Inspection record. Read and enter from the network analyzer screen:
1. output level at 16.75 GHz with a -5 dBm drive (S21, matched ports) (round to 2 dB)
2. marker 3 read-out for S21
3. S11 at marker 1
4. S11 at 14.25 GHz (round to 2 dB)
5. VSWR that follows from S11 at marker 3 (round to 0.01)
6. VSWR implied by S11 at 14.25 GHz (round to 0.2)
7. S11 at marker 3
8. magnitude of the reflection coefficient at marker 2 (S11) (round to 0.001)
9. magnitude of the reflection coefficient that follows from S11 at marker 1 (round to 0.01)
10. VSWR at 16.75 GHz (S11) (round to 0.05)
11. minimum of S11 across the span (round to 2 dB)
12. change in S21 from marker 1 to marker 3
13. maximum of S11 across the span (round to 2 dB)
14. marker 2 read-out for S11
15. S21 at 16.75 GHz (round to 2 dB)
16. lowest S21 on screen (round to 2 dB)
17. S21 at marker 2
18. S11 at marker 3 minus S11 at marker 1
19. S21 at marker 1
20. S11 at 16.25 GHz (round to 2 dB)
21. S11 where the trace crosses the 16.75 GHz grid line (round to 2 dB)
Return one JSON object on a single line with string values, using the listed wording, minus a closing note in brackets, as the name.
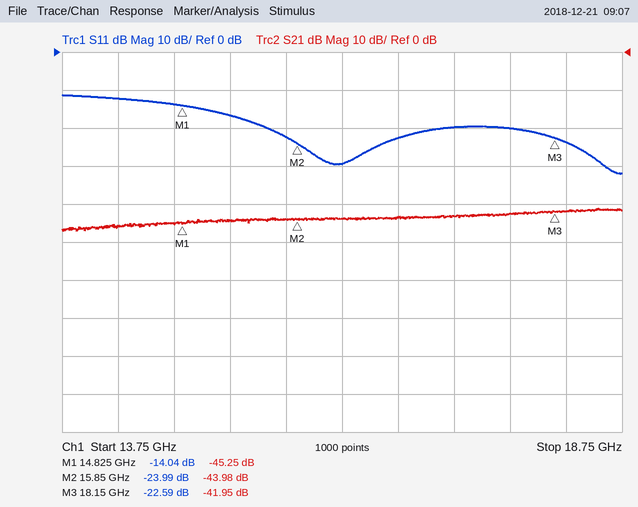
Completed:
{"output level at 16.75 GHz with a -5 dBm drive (S21, matched ports)": "-48 dBm", "marker 3 read-out for S21": "-41.95 dB", "S11 at marker 1": "-14.04 dB", "S11 at 14.25 GHz": "-12 dB", "VSWR that follows from S11 at marker 3": "1.16", "VSWR implied by S11 at 14.25 GHz": "1.6", "S11 at marker 3": "-22.59 dB", "magnitude of the reflection coefficient at marker 2 (S11)": "0.063", "magnitude of the reflection coefficient that follows from S11 at marker 1": "0.20", "VSWR at 16.75 GHz (S11)": "1.15", "minimum of S11 across the span": "-32 dB", "change in S21 from marker 1 to marker 3": "3.30 dB", "maximum of S11 across the span": "-12 dB", "marker 2 read-out for S11": "-23.99 dB", "S21 at 16.75 GHz": "-44 dB", "lowest S21 on screen": "-48 dB", "S21 at marker 2": "-43.98 dB", "S11 at marker 3 minus S11 at marker 1": "-8.55 dB", "S21 at marker 1": "-45.25 dB", "S11 at 16.25 GHz": "-30 dB", "S11 where the trace crosses the 16.75 GHz grid line": "-22 dB"}
